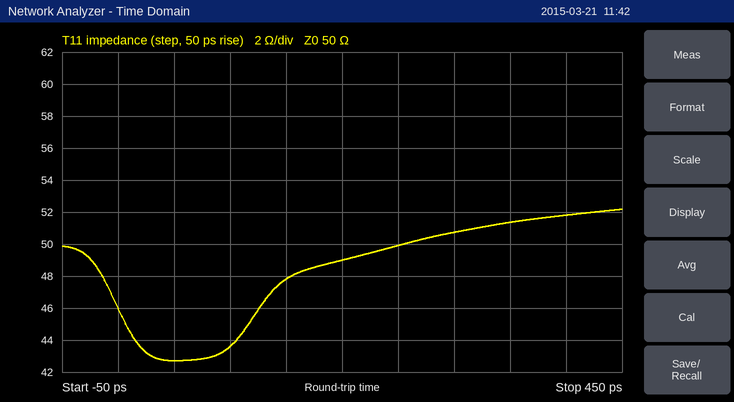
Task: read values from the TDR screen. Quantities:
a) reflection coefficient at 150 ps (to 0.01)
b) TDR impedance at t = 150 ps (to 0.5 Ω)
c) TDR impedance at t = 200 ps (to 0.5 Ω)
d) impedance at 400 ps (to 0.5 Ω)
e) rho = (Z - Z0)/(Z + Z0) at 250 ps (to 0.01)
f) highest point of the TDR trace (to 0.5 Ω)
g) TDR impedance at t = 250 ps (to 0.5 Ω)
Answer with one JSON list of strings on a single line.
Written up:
["-0.02", "48.0 Ω", "49.0 Ω", "52.0 Ω", "0.00", "52.0 Ω", "50.0 Ω"]
